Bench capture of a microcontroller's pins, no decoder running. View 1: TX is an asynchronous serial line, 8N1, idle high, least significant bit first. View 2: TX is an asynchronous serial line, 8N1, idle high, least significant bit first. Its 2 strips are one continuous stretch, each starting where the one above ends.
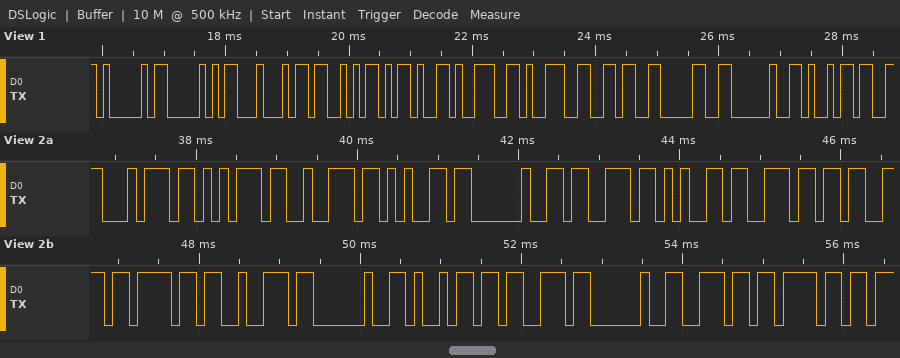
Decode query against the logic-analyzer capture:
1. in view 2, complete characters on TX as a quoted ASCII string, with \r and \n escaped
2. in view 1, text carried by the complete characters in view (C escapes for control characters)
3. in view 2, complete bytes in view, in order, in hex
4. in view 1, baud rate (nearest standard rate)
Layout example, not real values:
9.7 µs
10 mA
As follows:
"ture sensor is no"
"APDS-9960 i"
74 75 72 65 20 73 65 6E 73 6F 72 20 69 73 20 6E 6F
9600 baud
